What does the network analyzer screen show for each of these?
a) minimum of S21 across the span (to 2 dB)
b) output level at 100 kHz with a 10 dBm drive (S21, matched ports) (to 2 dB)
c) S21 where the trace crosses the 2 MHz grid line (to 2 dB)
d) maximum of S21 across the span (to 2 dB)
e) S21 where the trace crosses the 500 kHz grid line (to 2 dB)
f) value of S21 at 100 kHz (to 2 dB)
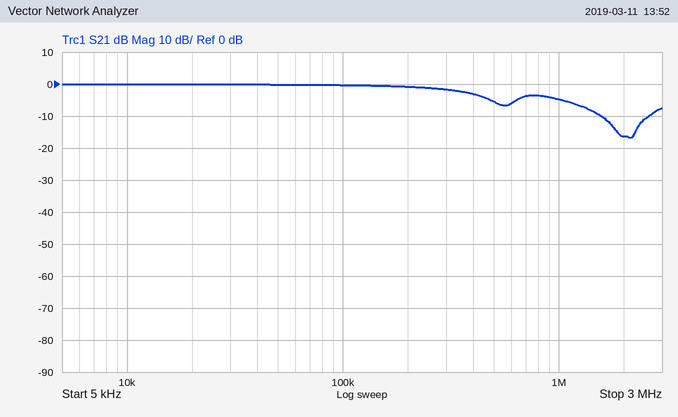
-16 dB
10 dBm
-16 dB
0 dB
-6 dB
0 dB
